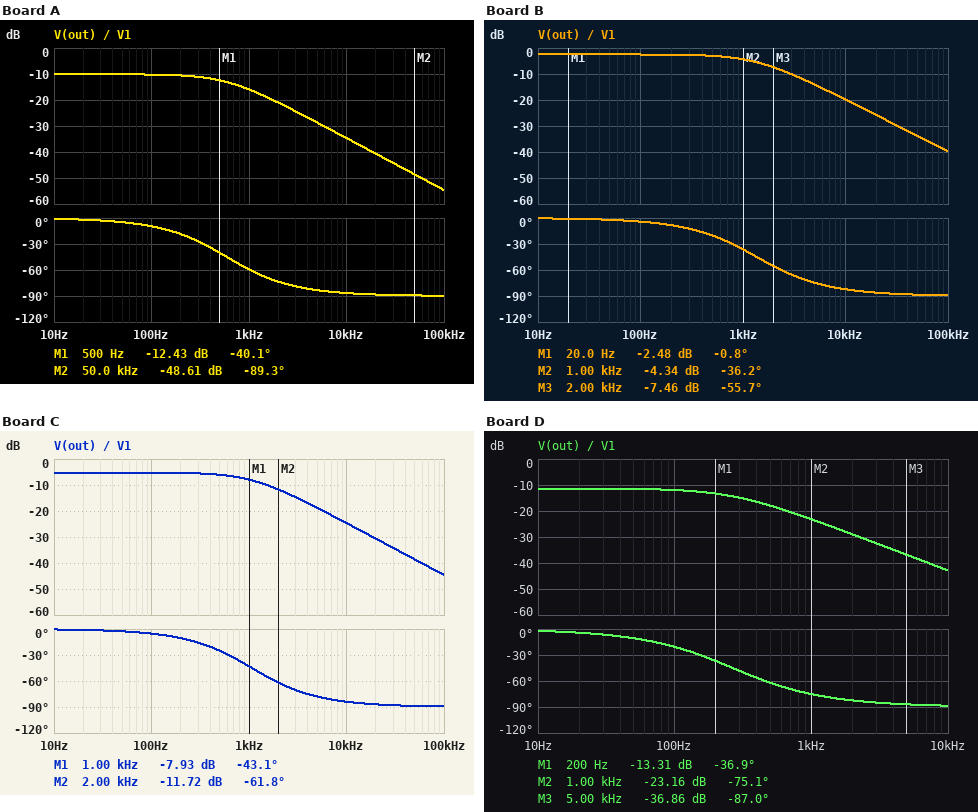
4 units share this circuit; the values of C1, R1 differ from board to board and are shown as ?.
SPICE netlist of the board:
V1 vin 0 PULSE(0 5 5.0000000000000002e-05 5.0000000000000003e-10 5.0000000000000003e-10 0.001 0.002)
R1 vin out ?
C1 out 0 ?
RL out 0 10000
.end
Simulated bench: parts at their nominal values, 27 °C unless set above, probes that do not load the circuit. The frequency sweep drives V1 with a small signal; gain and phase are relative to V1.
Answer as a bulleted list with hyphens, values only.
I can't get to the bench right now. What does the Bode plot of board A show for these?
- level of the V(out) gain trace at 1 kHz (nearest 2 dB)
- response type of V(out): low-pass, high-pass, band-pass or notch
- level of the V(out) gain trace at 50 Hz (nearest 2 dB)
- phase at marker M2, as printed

- -16 dB
- low-pass
- -10 dB
- -89.3 deg
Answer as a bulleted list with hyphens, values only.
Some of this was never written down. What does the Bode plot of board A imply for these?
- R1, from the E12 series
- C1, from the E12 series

- 22 kΩ
- 39 nF
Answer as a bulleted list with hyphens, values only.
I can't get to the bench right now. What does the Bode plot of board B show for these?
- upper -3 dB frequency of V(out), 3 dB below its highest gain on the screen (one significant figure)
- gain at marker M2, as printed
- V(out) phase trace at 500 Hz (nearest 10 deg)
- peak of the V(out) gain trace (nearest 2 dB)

- 1 kHz
- -4.34 dB
- -20 deg
- -2 dB
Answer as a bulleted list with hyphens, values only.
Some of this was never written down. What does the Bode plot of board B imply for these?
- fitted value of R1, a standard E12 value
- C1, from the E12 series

- 3.3 kΩ
- 47 nF
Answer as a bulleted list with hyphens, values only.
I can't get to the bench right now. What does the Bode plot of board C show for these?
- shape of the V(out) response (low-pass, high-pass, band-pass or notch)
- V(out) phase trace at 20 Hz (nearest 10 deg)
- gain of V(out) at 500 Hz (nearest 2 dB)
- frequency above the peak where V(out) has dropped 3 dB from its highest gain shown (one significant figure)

- low-pass
- 0 deg
- -6 dB
- 1 kHz
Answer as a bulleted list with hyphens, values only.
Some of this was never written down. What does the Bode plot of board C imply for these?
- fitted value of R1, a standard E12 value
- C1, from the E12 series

- 8.2 kΩ
- 33 nF
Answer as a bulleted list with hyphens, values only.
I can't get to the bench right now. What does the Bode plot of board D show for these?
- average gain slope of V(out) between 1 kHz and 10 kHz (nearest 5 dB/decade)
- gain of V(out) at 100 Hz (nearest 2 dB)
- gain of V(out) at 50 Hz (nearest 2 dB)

- -20 dB/decade
- -12 dB
- -12 dB
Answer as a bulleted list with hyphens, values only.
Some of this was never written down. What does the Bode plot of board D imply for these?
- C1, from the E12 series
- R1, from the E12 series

- 82 nF
- 27 kΩ
